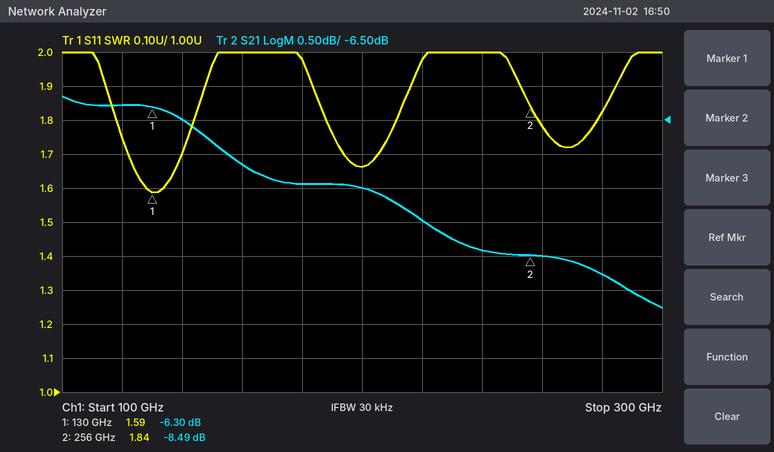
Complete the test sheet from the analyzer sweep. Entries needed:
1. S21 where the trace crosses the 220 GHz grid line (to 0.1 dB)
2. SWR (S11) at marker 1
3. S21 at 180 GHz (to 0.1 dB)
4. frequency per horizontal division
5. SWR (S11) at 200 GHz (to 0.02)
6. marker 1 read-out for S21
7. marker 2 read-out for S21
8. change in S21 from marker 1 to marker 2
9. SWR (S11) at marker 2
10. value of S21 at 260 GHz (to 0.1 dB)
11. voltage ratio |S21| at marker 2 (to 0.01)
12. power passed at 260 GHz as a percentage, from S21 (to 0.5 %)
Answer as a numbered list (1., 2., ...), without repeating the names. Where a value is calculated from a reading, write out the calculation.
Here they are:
1. -8.0 dB
2. 1.59
3. -7.4 dB
4. 20 GHz
5. 1.66
6. -6.30 dB
7. -8.49 dB
8. -8.49 − (-6.3) = -2.19 dB
9. 1.84
10. -8.5 dB
11. 10^(-8.49/20) ≈ 0.38
12. 10^(-8.5/10) ≈ 14.1 %, so 14.0 % to the nearest 0.5 %
